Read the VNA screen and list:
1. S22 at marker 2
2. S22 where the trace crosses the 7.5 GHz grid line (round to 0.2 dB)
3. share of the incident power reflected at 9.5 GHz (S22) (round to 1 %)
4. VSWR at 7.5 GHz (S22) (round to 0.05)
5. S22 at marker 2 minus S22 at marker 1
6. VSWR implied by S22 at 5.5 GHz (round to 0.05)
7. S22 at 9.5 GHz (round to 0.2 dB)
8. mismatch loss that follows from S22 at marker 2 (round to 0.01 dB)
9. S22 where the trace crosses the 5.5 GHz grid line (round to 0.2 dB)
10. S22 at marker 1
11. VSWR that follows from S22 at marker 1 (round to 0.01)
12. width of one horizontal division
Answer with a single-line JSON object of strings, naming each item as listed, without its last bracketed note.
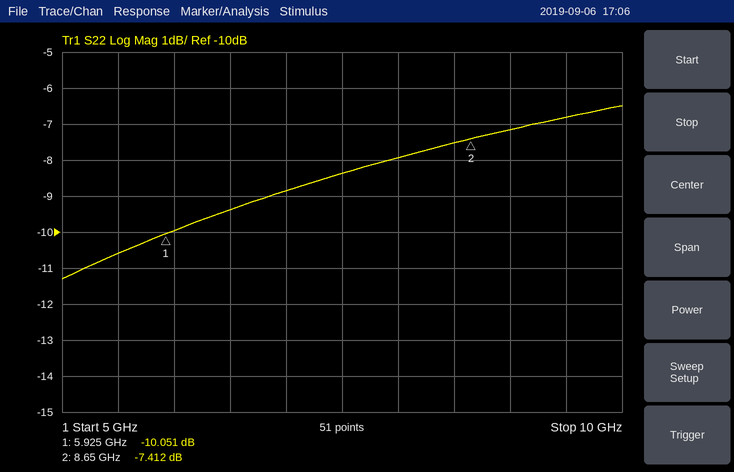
{"S22 at marker 2": "-7.412 dB", "S22 where the trace crosses the 7.5 GHz grid line": "-8.4 dB", "share of the incident power reflected at 9.5 GHz (S22)": "21 %", "VSWR at 7.5 GHz (S22)": "2.25", "S22 at marker 2 minus S22 at marker 1": "2.639 dB", "VSWR implied by S22 at 5.5 GHz": "1.85", "S22 at 9.5 GHz": "-6.8 dB", "mismatch loss that follows from S22 at marker 2": "0.87 dB", "S22 where the trace crosses the 5.5 GHz grid line": "-10.6 dB", "S22 at marker 1": "-10.051 dB", "VSWR that follows from S22 at marker 1": "1.92", "width of one horizontal division": "500 MHz"}
